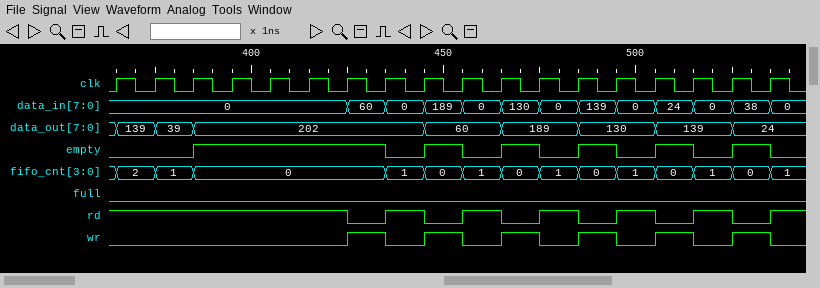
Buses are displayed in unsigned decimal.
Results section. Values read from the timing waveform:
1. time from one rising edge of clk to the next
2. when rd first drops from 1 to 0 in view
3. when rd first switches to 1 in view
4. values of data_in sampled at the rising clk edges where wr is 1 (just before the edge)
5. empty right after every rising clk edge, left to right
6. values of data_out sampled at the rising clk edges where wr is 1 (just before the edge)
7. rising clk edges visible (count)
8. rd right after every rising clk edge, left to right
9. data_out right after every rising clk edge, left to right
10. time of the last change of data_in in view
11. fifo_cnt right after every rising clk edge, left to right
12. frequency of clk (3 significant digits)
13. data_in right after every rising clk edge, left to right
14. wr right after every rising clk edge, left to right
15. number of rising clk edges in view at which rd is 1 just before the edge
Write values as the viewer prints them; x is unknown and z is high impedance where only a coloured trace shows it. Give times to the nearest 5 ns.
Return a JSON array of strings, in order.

["10 ns", "425 ns", "435 ns", "60, 189, 130, 139, 24, 38", "0 0 1 1 1 1 1 0 1 0 1 0 1 0 1 0 1 0", "202, 60, 189, 130, 139, 24", "18", "1 1 1 1 1 1 0 1 0 1 0 1 0 1 0 1 0 1", "139, 39, 202, 202, 202, 202, 202, 202, 60, 60, 189, 189, 130, 130, 139, 139, 24, 24", "535 ns", "2, 1, 0, 0, 0, 0, 0, 1, 0, 1, 0, 1, 0, 1, 0, 1, 0, 1", "100 MHz", "0, 0, 0, 0, 0, 0, 60, 0, 189, 0, 130, 0, 139, 0, 24, 0, 38, 0", "0 0 0 0 0 0 1 0 1 0 1 0 1 0 1 0 1 0", "12"]
